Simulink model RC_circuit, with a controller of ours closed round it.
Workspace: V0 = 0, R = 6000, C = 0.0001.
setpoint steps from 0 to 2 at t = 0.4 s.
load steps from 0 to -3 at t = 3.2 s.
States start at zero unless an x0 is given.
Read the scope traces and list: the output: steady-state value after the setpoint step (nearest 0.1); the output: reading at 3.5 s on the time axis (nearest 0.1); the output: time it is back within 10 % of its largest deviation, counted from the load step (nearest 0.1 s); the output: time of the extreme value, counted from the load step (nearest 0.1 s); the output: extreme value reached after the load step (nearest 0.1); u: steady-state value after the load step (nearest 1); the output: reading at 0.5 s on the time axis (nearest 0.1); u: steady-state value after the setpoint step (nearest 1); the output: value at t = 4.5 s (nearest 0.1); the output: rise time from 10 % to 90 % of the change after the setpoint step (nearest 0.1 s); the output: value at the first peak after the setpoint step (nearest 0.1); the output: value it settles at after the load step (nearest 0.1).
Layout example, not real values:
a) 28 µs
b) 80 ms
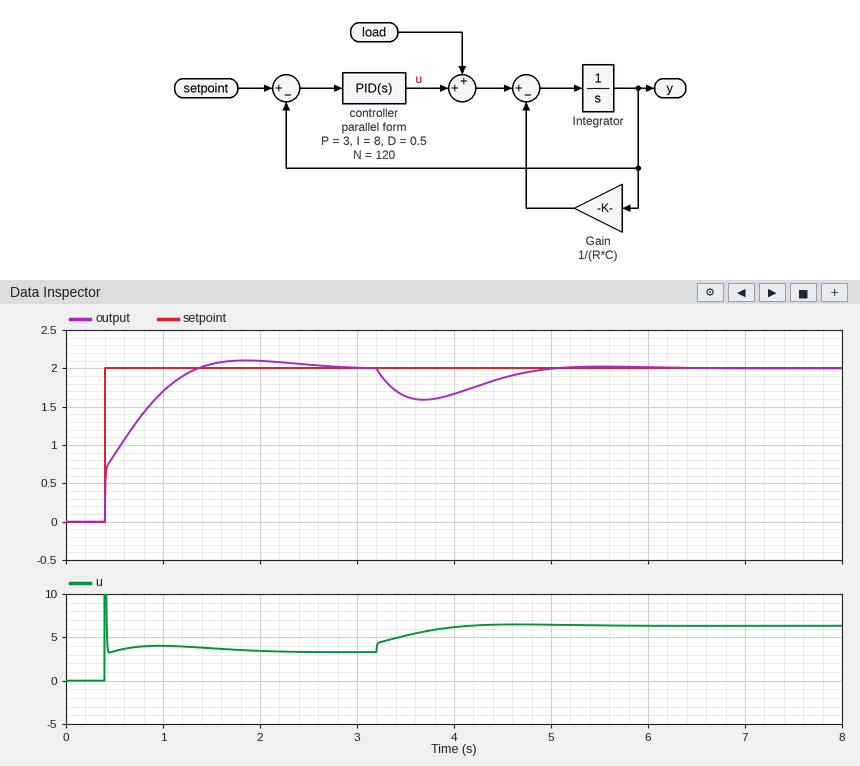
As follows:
a) 2.0
b) 1.6
c) 1.6 s
d) 0.5 s
e) 1.6
f) 6
g) 0.9
h) 3
i) 1.9
j) 0.7 s
k) 2.1
l) 2.0
